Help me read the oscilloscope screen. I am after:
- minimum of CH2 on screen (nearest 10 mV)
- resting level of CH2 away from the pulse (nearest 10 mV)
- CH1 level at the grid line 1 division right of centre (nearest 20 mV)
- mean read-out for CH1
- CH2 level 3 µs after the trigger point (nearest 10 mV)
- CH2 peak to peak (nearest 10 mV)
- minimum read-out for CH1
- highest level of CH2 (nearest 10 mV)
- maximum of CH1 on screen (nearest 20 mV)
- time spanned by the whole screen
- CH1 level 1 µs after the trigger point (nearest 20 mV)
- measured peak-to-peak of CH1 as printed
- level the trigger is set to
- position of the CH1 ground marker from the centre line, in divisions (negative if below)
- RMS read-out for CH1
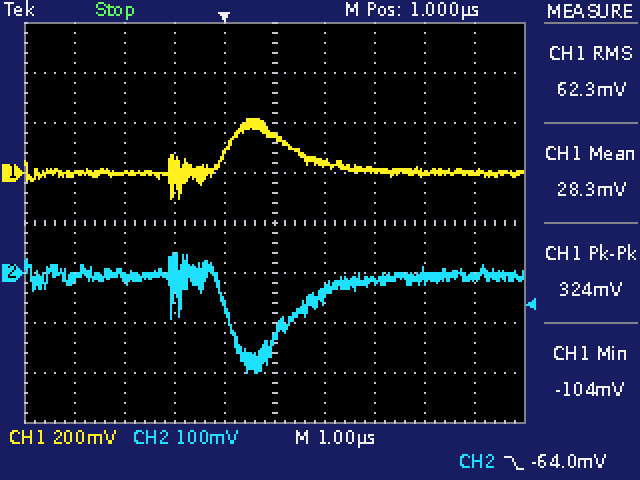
-200 mV
-10 mV
40 mV
28.3 mV
-20 mV
240 mV
-104 mV
40 mV
220 mV
10 µs
140 mV
324 mV
-64.0 mV
+1.0 div
62.3 mV
